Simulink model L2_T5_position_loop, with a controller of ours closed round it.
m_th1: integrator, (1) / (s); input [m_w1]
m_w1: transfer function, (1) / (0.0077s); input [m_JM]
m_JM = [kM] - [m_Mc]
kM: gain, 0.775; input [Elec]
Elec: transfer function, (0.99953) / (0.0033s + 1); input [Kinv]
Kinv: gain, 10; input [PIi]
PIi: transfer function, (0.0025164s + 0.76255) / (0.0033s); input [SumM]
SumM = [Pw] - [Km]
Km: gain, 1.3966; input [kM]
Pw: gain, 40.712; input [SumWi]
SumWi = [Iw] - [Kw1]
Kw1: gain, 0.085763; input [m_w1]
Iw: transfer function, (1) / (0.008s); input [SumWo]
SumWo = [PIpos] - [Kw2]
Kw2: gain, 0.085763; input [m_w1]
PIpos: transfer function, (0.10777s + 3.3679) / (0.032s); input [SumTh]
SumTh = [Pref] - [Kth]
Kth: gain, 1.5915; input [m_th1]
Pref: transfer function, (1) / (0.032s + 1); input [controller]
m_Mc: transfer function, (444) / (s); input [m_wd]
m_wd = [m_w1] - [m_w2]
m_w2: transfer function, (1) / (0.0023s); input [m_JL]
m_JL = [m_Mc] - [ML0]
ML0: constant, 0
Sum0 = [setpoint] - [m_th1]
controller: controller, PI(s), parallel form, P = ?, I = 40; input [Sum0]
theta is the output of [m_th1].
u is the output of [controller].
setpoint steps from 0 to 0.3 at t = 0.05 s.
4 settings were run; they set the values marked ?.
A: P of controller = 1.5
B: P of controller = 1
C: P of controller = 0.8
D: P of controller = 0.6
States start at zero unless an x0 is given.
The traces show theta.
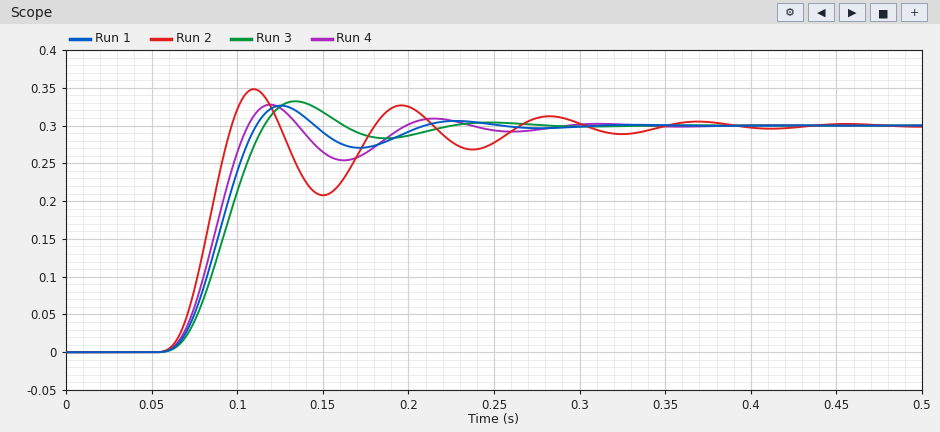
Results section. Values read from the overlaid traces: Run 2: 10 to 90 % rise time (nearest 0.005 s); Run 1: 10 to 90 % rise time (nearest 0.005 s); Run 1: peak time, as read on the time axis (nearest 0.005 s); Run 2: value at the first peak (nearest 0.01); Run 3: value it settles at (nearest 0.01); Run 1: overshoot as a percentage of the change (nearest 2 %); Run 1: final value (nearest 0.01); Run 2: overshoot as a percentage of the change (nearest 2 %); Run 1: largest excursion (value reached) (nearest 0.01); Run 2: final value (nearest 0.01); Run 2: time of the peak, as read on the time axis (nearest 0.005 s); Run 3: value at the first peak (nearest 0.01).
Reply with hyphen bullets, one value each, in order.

- 0.025 s
- 0.035 s
- 0.125 s
- 0.35
- 0.30
- 8 %
- 0.30
- 16 %
- 0.33
- 0.30
- 0.110 s
- 0.33
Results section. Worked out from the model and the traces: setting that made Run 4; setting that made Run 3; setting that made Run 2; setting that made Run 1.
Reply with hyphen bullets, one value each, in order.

- B
- D
- A
- C
